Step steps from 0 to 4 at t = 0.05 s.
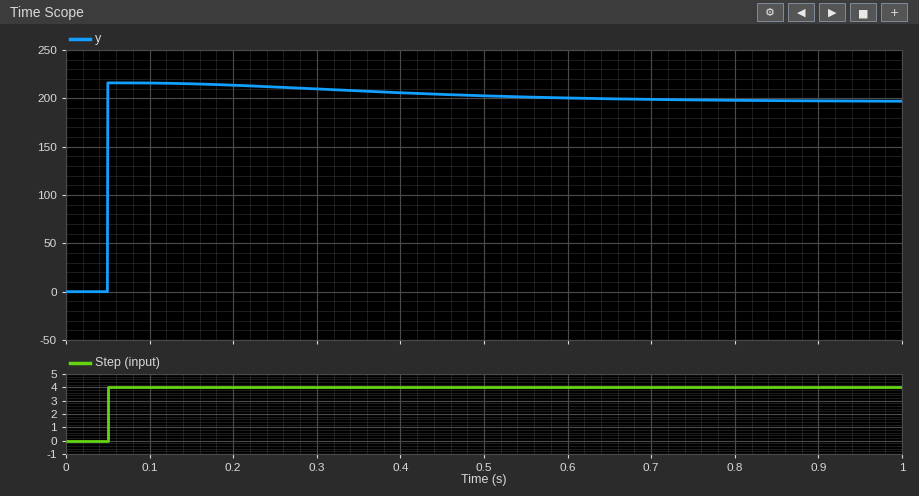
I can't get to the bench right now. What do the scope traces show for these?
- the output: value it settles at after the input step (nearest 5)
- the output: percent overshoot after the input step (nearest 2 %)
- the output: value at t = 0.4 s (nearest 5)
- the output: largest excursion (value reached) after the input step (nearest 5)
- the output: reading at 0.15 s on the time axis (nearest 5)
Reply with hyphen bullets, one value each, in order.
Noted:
- 195
- 10 %
- 205
- 215
- 215
